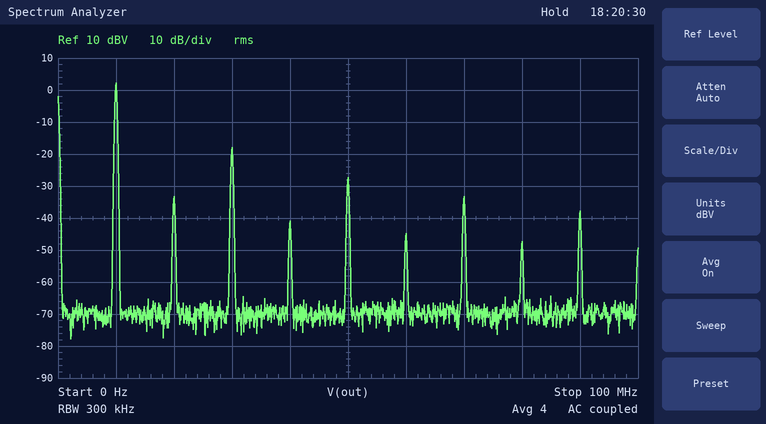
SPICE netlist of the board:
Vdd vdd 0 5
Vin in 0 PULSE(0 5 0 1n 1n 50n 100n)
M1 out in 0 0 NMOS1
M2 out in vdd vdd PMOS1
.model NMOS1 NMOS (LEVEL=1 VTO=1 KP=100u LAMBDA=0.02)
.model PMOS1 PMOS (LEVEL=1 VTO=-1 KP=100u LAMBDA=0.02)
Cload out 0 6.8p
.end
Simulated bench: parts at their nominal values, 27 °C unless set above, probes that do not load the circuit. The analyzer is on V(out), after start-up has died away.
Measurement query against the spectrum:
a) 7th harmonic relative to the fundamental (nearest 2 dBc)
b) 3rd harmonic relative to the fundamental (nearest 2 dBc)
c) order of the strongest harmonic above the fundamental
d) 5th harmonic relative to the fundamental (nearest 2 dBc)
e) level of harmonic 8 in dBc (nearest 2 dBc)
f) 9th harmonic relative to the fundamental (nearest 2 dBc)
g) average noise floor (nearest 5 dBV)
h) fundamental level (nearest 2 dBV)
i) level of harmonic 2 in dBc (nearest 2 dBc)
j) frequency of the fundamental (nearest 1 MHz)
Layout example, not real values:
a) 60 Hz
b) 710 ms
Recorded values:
a) -36 dBc
b) -20 dBc
c) 3
d) -30 dBc
e) -50 dBc
f) -40 dBc
g) -70 dBV
h) 2 dBV
i) -36 dBc
j) 10 MHz
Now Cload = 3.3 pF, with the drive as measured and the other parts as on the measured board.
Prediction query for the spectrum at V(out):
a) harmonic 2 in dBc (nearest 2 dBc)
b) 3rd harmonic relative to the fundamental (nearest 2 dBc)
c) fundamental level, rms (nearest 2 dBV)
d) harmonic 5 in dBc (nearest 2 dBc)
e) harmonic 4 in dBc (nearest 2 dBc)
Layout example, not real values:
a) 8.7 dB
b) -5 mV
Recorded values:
a) -34 dBc
b) -16 dBc
c) 6 dBV
d) -28 dBc
e) -40 dBc
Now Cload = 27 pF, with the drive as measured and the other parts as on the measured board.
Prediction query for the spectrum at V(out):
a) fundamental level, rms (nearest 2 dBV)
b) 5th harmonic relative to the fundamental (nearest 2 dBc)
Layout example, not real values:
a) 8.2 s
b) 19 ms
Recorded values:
a) -8 dBV
b) -28 dBc
